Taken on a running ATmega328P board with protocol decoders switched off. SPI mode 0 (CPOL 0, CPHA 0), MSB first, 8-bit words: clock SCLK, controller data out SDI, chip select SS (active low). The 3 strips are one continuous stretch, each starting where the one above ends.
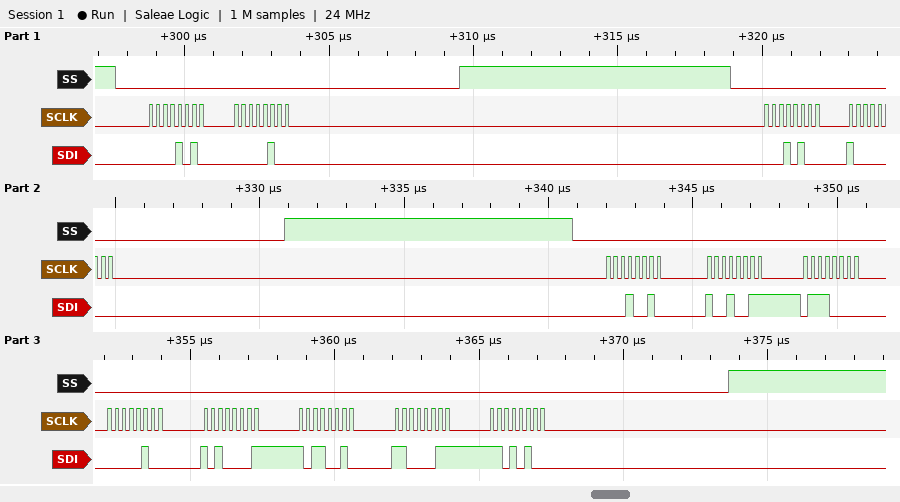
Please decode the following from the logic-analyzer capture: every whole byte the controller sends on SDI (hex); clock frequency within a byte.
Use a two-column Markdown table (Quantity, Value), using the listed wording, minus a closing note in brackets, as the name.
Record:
| Quantity | Value |
|---|---|
| every whole byte the controller sends on SDI | 0A 04 14 80 12 93 70 04 A1 B2 C3 D4 |
| clock frequency within a byte | 4 MHz |
